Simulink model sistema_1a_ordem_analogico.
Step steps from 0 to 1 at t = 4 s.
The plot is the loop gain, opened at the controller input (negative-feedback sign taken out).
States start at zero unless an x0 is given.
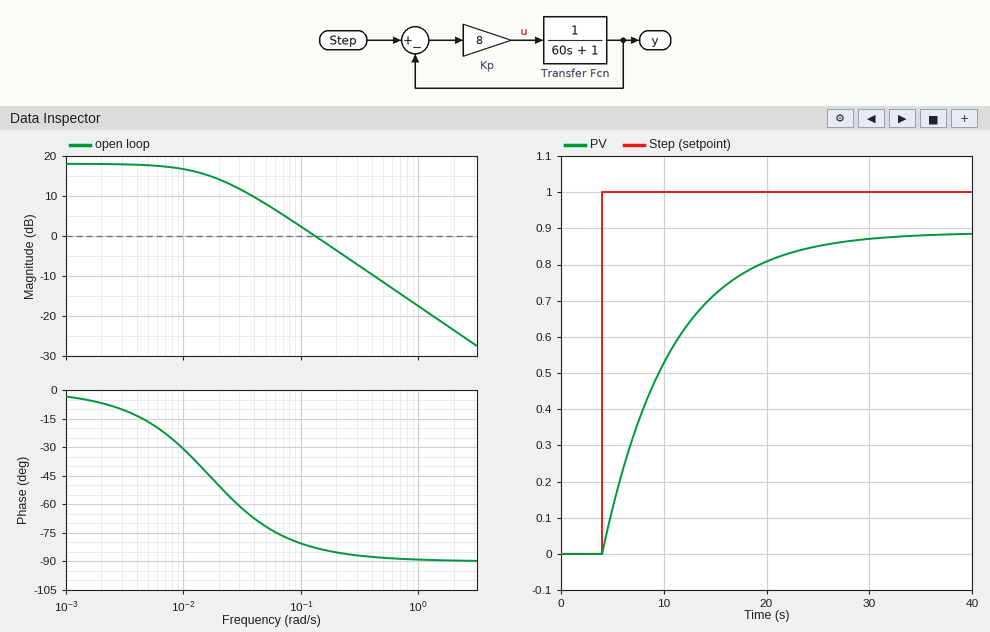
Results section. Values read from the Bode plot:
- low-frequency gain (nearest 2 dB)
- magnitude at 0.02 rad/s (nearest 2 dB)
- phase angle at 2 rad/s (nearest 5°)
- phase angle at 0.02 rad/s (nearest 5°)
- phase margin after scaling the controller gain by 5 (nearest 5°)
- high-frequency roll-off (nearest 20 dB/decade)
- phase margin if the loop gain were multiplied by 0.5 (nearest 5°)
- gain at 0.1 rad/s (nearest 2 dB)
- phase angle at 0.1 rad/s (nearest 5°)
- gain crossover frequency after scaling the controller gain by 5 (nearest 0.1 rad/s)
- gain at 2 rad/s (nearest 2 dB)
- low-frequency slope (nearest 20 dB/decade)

18 dB
14 dB
-90°
-50°
90°
-20 dB/decade
105°
2 dB
-80°
0.7 rad/s
-24 dB
0 dB/decade
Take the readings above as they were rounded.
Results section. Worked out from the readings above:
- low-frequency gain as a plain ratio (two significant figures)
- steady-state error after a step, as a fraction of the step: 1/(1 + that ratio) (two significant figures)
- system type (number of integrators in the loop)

7.9
0.11
0
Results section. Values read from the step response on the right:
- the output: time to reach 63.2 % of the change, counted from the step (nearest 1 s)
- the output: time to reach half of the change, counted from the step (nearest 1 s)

7 s
5 s
